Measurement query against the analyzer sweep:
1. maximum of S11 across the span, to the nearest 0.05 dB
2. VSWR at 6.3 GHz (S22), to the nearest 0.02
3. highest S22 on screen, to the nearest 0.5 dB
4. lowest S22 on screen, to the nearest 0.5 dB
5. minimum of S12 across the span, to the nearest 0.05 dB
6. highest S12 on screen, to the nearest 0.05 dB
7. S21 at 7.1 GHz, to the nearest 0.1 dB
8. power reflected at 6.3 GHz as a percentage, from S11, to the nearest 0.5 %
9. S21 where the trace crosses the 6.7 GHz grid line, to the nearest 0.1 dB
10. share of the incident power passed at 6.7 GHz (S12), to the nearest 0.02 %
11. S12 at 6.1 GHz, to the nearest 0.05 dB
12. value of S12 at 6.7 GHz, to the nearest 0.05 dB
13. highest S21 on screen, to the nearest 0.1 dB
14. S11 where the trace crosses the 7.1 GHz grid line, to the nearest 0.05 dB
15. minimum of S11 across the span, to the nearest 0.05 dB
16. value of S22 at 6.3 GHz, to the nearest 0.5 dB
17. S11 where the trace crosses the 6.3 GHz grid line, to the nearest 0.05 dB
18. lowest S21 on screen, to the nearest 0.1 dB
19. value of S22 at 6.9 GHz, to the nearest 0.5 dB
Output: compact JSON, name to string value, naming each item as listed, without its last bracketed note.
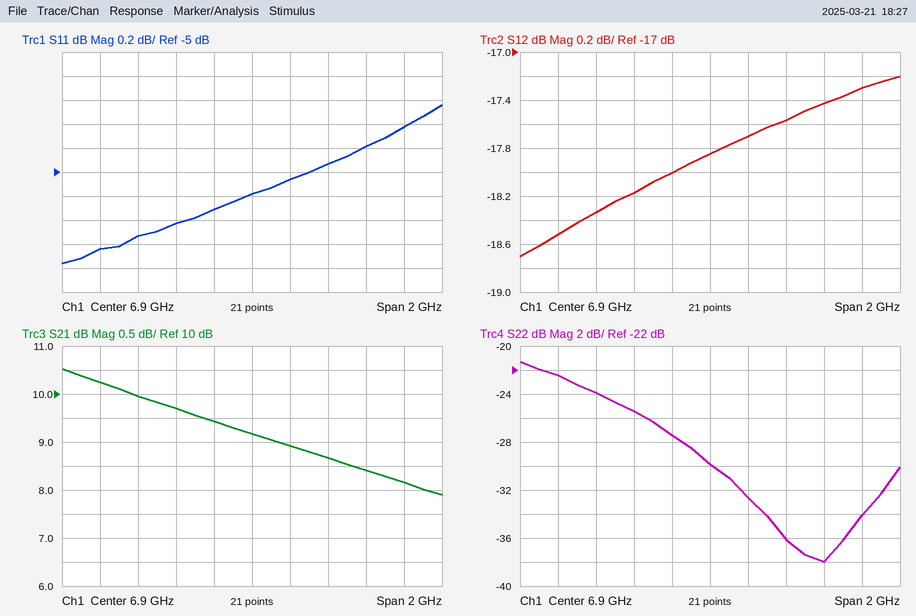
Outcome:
{"maximum of S11 across the span, to the nearest 0.05 dB": "-4.45 dB", "VSWR at 6.3 GHz (S22), to the nearest 0.02": "1.14", "highest S22 on screen, to the nearest 0.5 dB": "-21.5 dB", "lowest S22 on screen, to the nearest 0.5 dB": "-38.0 dB", "minimum of S12 across the span, to the nearest 0.05 dB": "-18.70 dB", "highest S12 on screen, to the nearest 0.05 dB": "-17.20 dB", "S21 at 7.1 GHz, to the nearest 0.1 dB": "8.9 dB", "power reflected at 6.3 GHz as a percentage, from S11, to the nearest 0.5 %": "28.0 %", "S21 where the trace crosses the 6.7 GHz grid line, to the nearest 0.1 dB": "9.4 dB", "share of the incident power passed at 6.7 GHz (S12), to the nearest 0.02 %": "1.58 %", "S12 at 6.1 GHz, to the nearest 0.05 dB": "-18.50 dB", "value of S12 at 6.7 GHz, to the nearest 0.05 dB": "-18.00 dB", "highest S21 on screen, to the nearest 0.1 dB": "10.5 dB", "S11 where the trace crosses the 7.1 GHz grid line, to the nearest 0.05 dB": "-5.05 dB", "minimum of S11 across the span, to the nearest 0.05 dB": "-5.75 dB", "value of S22 at 6.3 GHz, to the nearest 0.5 dB": "-24.0 dB", "S11 where the trace crosses the 6.3 GHz grid line, to the nearest 0.05 dB": "-5.55 dB", "lowest S21 on screen, to the nearest 0.1 dB": "7.9 dB", "value of S22 at 6.9 GHz, to the nearest 0.5 dB": "-30.0 dB"}
